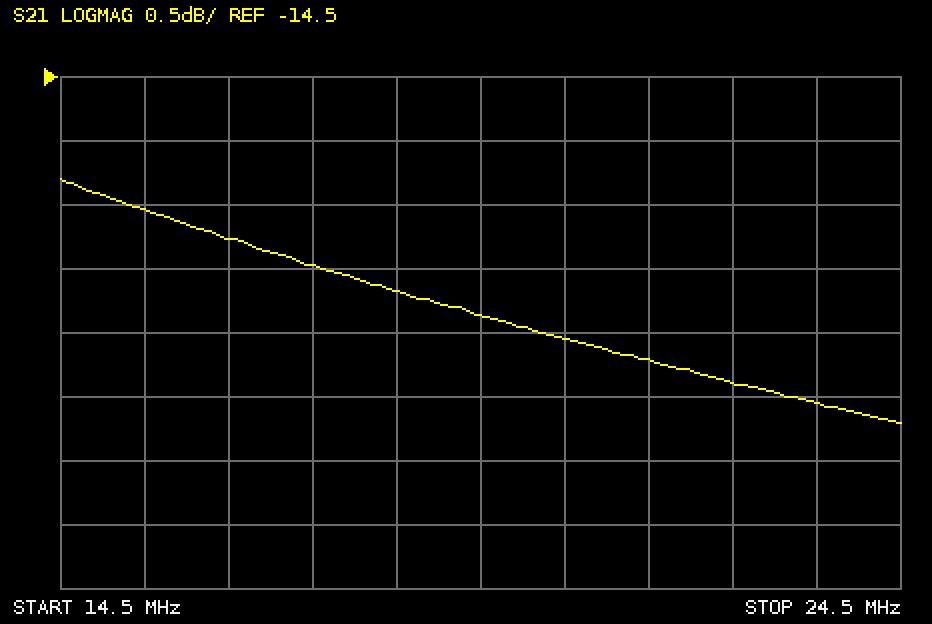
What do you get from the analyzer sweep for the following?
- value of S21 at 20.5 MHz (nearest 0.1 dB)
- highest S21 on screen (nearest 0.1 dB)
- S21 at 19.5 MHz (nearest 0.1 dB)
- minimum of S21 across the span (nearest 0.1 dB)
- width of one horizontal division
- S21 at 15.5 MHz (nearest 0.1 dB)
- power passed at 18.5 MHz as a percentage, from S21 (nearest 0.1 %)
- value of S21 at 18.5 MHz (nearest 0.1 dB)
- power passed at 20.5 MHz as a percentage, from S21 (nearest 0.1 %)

-16.5 dB
-15.3 dB
-16.4 dB
-17.2 dB
1 MHz
-15.5 dB
2.4 %
-16.2 dB
2.2 %
